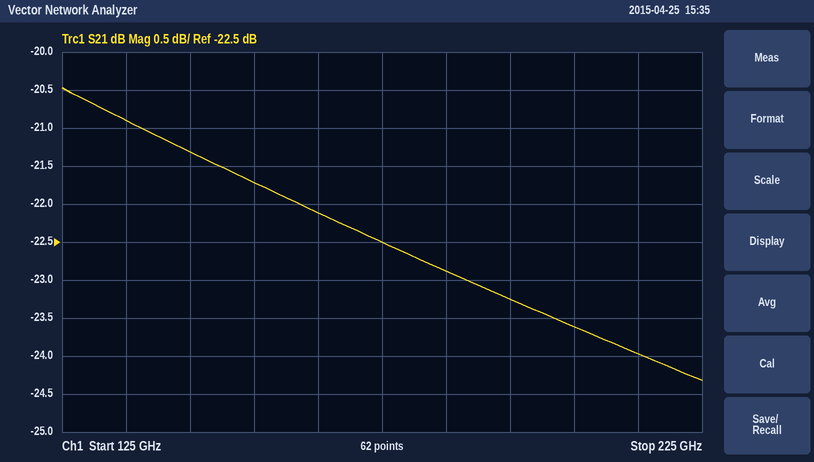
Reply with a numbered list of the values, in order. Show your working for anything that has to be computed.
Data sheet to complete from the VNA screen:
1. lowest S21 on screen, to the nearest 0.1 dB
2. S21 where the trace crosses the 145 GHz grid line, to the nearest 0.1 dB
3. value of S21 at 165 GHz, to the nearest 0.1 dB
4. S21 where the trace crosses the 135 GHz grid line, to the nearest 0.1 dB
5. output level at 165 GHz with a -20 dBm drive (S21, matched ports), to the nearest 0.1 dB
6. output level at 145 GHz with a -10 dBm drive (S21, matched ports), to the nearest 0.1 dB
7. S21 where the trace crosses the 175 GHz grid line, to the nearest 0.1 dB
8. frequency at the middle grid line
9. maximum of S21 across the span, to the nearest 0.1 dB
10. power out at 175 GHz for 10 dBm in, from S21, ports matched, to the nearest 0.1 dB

1. -24.3 dB
2. -21.3 dB
3. -22.1 dB
4. -20.9 dB
5. -20 dBm + (-22.1 dB) = -42.1 dBm
6. -10 dBm + (-21.3 dB) = -31.3 dBm
7. -22.5 dB
8. 175 GHz
9. -20.5 dB
10. 10 dBm + (-22.5 dB) = -12.5 dBm
